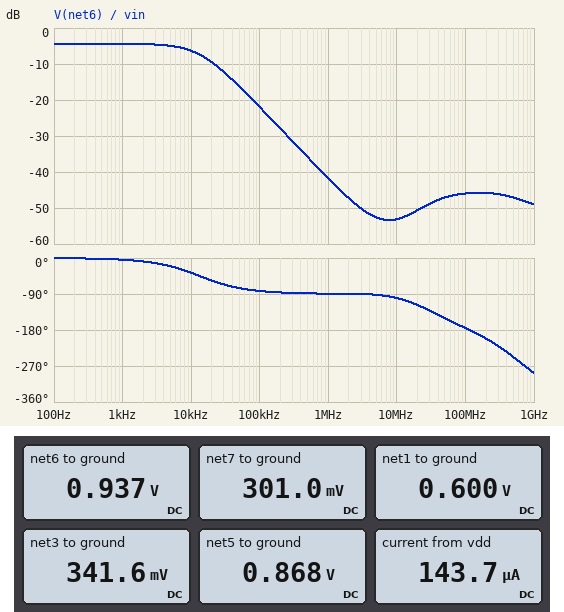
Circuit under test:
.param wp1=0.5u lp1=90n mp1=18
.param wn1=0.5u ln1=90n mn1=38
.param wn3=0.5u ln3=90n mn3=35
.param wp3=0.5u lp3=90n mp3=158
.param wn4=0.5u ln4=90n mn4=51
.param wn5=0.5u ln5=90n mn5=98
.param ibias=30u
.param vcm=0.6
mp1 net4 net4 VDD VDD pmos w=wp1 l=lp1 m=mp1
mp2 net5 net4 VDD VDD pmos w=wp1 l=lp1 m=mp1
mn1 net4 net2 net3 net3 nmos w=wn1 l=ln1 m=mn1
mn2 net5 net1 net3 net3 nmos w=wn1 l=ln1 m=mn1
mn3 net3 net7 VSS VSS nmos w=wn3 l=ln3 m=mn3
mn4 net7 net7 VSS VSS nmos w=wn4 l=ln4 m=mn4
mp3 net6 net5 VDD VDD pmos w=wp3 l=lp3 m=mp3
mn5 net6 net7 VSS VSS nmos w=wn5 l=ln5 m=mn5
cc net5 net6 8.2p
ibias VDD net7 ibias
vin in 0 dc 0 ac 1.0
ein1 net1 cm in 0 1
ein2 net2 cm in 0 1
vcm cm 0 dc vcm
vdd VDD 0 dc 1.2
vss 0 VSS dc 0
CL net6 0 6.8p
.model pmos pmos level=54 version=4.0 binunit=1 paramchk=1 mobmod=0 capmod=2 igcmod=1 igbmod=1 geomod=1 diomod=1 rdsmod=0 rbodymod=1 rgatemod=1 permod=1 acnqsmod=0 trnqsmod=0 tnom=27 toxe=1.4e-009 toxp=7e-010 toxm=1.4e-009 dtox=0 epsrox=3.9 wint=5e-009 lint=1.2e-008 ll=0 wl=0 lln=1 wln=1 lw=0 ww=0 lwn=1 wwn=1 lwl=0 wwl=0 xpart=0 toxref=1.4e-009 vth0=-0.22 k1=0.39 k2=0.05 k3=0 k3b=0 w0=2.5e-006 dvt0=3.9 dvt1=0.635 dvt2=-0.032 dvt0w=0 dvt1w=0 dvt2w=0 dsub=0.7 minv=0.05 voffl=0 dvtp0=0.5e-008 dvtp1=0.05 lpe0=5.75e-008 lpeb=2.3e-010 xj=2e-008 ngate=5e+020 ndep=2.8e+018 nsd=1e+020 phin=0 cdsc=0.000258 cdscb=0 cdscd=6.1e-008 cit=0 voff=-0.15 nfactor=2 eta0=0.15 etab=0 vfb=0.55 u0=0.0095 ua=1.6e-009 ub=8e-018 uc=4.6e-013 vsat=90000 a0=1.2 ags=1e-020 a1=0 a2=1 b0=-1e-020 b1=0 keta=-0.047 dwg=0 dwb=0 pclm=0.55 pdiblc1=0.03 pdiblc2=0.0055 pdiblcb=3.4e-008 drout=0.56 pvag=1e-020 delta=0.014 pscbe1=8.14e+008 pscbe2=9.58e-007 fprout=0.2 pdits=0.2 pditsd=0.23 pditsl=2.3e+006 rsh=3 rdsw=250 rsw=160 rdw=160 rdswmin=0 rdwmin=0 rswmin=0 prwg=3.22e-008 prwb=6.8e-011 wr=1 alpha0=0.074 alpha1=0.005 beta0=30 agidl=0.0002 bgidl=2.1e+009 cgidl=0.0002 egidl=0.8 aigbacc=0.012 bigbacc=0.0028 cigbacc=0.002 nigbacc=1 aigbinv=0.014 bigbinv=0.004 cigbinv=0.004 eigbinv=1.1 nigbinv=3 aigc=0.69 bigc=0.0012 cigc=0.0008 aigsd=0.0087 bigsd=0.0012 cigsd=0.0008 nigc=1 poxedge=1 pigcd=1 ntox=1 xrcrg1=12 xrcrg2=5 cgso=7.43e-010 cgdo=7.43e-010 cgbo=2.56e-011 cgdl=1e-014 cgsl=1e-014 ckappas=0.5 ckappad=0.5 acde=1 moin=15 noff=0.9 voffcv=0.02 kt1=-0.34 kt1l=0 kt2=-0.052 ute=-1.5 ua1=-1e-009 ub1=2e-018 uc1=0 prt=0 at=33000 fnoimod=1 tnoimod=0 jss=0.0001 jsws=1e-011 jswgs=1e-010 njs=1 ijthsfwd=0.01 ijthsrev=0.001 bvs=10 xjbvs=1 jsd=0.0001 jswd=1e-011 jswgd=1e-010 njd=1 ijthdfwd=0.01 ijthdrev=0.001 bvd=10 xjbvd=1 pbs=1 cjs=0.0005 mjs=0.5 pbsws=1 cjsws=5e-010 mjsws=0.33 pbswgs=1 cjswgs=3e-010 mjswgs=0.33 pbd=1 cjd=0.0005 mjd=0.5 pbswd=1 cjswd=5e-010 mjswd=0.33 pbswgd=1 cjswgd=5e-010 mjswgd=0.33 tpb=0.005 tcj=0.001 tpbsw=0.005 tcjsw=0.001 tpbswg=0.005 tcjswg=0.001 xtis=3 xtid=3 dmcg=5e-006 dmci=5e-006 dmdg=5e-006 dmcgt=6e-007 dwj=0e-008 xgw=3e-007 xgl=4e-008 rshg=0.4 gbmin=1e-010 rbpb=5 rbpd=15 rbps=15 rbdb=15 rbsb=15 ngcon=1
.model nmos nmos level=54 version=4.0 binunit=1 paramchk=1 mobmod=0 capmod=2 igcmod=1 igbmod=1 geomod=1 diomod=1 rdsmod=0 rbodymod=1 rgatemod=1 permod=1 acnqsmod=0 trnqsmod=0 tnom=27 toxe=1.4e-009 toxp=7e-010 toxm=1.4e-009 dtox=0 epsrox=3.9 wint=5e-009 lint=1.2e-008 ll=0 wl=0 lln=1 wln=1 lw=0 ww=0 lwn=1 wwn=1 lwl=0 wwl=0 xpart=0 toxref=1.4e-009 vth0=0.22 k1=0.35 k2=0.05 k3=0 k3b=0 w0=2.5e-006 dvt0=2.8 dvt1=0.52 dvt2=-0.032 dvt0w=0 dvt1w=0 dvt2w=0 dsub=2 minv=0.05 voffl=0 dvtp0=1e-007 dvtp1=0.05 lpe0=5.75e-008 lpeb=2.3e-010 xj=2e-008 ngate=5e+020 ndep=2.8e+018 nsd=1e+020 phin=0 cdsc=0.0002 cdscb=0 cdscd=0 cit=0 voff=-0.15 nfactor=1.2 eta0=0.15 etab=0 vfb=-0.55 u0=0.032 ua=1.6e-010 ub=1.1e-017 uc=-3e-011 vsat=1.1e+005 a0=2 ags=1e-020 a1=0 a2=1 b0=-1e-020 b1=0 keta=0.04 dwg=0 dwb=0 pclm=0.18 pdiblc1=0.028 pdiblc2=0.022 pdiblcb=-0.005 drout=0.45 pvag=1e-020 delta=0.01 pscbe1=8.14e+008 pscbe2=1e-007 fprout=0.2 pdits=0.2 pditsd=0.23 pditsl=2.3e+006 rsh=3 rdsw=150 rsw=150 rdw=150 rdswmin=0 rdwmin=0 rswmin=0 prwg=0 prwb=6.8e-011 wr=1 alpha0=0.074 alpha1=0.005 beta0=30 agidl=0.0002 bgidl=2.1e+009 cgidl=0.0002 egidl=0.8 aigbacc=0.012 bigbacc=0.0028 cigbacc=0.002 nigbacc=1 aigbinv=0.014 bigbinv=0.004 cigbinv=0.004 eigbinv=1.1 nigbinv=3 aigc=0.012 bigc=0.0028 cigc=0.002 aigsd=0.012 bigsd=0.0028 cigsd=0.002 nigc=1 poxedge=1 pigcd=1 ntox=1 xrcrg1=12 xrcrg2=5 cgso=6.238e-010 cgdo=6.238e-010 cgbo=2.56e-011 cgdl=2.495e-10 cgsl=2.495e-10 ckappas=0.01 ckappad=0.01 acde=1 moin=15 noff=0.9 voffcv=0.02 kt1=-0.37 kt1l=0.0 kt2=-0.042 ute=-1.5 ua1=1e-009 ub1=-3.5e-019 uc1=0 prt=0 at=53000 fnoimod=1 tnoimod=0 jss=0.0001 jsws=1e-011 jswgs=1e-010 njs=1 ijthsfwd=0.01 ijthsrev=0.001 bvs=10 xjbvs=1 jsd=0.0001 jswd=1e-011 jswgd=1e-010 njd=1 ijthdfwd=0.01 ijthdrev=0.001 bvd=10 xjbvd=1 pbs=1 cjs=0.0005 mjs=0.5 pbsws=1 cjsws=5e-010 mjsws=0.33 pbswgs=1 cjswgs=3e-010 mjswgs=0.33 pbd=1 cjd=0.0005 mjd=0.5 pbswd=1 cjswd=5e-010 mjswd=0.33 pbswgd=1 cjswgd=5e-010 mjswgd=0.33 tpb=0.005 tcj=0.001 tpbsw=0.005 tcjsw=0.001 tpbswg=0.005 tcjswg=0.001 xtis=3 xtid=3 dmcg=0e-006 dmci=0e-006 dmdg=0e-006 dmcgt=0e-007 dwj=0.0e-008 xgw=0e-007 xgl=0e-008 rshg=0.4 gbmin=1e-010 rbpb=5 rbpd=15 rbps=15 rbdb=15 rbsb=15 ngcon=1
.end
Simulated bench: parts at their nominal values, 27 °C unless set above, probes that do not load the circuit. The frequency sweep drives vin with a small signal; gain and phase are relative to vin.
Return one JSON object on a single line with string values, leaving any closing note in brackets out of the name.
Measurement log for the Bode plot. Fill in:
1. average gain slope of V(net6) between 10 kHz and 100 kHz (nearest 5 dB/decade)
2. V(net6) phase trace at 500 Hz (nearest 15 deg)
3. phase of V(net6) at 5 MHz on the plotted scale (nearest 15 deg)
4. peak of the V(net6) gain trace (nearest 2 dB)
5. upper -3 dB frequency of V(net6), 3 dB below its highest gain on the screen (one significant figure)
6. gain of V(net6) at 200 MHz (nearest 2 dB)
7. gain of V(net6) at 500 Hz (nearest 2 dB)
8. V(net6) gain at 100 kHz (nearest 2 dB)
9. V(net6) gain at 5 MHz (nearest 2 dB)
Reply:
{"average gain slope of V(net6) between 10 kHz and 100 kHz": "-15 dB/decade", "V(net6) phase trace at 500 Hz": "0 deg", "phase of V(net6) at 5 MHz on the plotted scale": "-90 deg", "peak of the V(net6) gain trace": "-4 dB", "upper -3 dB frequency of V(net6), 3 dB below its highest gain on the screen": "10 kHz", "gain of V(net6) at 200 MHz": "-46 dB", "gain of V(net6) at 500 Hz": "-4 dB", "V(net6) gain at 100 kHz": "-22 dB", "V(net6) gain at 5 MHz": "-52 dB"}
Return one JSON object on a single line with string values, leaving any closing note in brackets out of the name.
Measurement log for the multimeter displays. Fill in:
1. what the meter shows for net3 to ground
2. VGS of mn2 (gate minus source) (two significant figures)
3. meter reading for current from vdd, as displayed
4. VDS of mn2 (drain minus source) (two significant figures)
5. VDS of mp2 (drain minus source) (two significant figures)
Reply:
{"what the meter shows for net3 to ground": "341.6 mV", "VGS of mn2 (gate minus source)": "260 mV", "meter reading for current from vdd, as displayed": "143.7 µA", "VDS of mn2 (drain minus source)": "530 mV", "VDS of mp2 (drain minus source)": "-330 mV"}
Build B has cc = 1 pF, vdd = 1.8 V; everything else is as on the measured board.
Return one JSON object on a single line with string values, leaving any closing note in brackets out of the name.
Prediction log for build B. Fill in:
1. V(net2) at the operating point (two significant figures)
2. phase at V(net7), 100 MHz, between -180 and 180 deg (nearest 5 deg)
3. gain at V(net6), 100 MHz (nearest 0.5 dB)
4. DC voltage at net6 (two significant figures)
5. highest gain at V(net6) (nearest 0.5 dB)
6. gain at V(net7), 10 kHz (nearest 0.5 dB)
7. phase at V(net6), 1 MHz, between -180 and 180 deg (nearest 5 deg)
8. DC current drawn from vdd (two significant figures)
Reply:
{"V(net2) at the operating point": "600 mV", "phase at V(net7), 100 MHz, between -180 and 180 deg": "80 deg", "gain at V(net6), 100 MHz": "-46.5 dB", "DC voltage at net6": "1.3 V", "highest gain at V(net6)": "-26.0 dB", "gain at V(net7), 10 kHz": "-51.0 dB", "phase at V(net6), 1 MHz, between -180 and 180 deg": "105 deg", "DC current drawn from vdd": "210 µA"}
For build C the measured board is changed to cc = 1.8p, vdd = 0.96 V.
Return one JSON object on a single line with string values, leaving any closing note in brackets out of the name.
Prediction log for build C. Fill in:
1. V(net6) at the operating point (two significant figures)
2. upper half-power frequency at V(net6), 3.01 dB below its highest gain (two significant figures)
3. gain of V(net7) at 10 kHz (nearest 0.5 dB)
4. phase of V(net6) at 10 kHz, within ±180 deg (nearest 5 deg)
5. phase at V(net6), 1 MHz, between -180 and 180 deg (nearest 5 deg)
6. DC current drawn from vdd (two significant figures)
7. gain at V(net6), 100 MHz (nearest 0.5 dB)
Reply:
{"V(net6) at the operating point": "810 mV", "upper half-power frequency at V(net6), 3.01 dB below its highest gain": "80 kHz", "gain of V(net7) at 10 kHz": "-49.0 dB", "phase of V(net6) at 10 kHz, within ±180 deg": "-5 deg", "phase at V(net6), 1 MHz, between -180 and 180 deg": "-85 deg", "DC current drawn from vdd": "130 µA", "gain at V(net6), 100 MHz": "-45.5 dB"}
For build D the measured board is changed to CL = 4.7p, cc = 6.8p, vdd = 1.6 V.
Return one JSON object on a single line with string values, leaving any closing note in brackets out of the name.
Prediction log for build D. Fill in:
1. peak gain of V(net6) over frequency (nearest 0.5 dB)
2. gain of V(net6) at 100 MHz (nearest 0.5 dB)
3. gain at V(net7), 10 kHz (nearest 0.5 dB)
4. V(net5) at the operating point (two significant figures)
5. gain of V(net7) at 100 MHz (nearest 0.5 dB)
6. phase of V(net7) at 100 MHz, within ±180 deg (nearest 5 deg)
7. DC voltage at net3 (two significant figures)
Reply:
{"peak gain of V(net6) over frequency": "-11.0 dB", "gain of V(net6) at 100 MHz": "-44.0 dB", "gain at V(net7), 10 kHz": "-41.0 dB", "V(net5) at the operating point": "1.3 V", "gain of V(net7) at 100 MHz": "-39.0 dB", "phase of V(net7) at 100 MHz, within ±180 deg": "80 deg", "DC voltage at net3": "350 mV"}
